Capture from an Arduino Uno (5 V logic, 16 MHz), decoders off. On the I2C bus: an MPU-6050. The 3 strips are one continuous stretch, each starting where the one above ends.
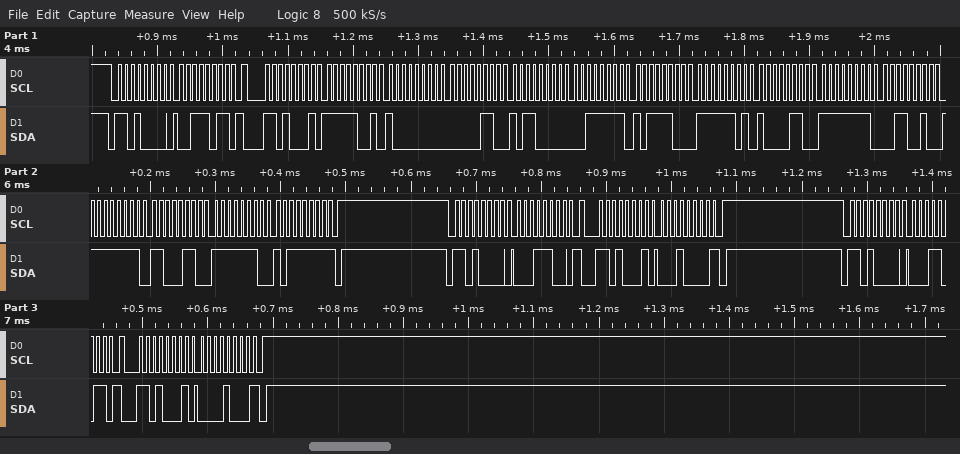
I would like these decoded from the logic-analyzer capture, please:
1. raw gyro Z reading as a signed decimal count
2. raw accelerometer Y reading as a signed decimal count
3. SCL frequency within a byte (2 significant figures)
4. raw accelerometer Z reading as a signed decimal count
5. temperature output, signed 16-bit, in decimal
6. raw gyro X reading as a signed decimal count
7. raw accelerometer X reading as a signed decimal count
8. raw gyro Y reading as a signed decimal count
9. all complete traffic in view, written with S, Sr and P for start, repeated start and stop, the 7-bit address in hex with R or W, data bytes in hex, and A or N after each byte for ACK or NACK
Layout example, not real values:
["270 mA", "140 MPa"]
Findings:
["-321", "1712", "100 kHz", "16316", "-634", "-206", "-1664", "-58", "S 68W A 3B A Sr 68R A F9 A 80 A 06 A B0 A 3F A BC A FD A 86 A FF A 32 A FF A C6 A FE A BF N P S 68W A 1C A Sr 68R A 10 N P S 68W A 1B A Sr 68R A 08 N P"]
